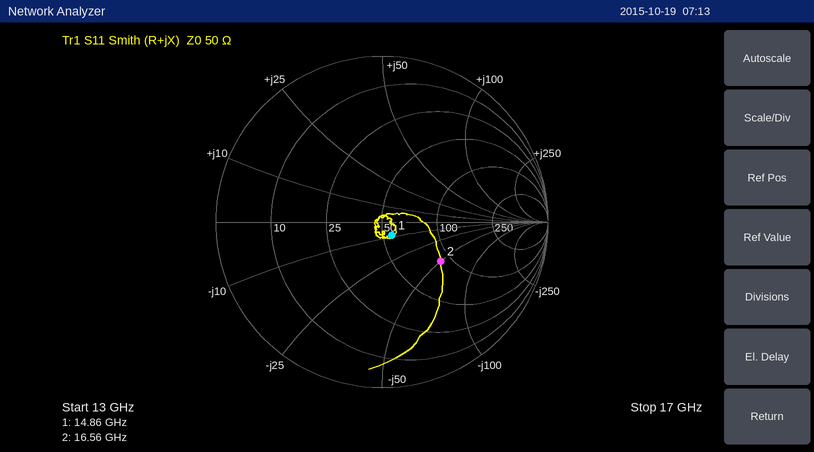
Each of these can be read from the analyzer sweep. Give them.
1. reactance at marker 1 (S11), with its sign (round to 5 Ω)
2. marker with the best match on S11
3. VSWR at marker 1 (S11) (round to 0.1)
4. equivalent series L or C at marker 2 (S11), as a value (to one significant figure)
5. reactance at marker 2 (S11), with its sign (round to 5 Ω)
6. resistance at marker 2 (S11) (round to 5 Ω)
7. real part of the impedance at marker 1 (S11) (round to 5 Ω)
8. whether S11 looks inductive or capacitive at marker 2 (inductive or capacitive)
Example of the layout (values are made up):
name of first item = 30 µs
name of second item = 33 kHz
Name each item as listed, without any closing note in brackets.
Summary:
reactance at marker 1 (S11), with its sign = -10 Ω
marker with the best match on S11 = marker 1
VSWR at marker 1 (S11) = 1.2
equivalent series L or C at marker 2 (S11), as a value = 200 fF
reactance at marker 2 (S11), with its sign = -50 Ω
resistance at marker 2 (S11) = 85 Ω
real part of the impedance at marker 1 (S11) = 55 Ω
whether S11 looks inductive or capacitive at marker 2 = capacitive
